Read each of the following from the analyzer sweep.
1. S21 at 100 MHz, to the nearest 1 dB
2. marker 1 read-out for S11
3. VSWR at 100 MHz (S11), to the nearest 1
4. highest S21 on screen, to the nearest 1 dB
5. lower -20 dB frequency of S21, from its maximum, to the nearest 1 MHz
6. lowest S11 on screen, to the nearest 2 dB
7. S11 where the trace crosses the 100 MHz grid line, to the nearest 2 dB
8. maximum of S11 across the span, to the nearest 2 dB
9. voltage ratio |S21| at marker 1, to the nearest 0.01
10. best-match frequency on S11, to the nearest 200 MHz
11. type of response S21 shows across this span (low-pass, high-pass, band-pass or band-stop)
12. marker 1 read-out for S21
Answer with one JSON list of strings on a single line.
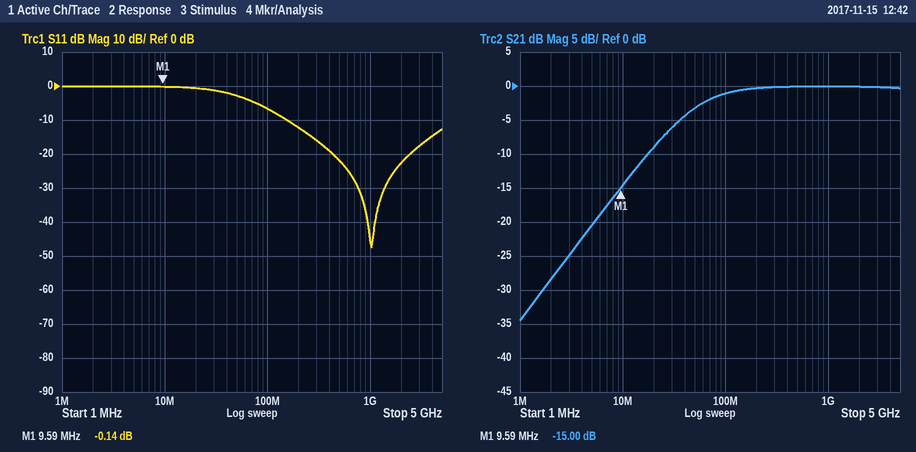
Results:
["-1 dB", "-0.14 dB", "3", "0 dB", "5 MHz", "-48 dB", "-6 dB", "0 dB", "0.18", "1.0 GHz", "high-pass", "-15.00 dB"]
